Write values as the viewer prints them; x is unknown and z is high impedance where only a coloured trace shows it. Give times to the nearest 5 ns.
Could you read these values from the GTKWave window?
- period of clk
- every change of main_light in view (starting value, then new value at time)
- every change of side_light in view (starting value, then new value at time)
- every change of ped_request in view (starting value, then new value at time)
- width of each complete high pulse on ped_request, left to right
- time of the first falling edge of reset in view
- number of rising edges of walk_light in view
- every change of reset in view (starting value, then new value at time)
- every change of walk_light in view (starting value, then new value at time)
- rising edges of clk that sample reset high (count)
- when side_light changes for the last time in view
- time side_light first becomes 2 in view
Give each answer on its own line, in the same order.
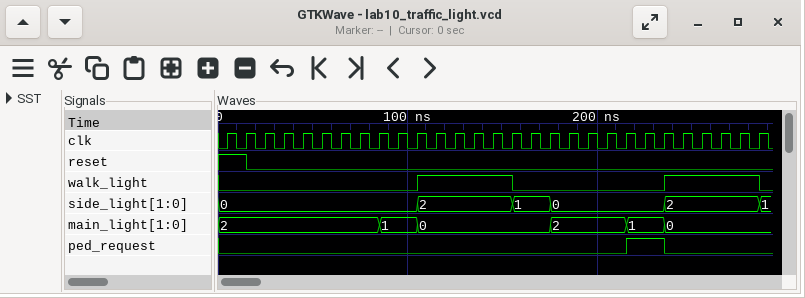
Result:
10 ns
2, 1 at 85 ns, 0 at 105 ns, 2 at 175 ns, 1 at 215 ns, 0 at 235 ns
0, 2 at 105 ns, 1 at 155 ns, 0 at 175 ns, 2 at 235 ns, 1 at 285 ns
0, 1 at 215 ns, 0 at 235 ns
20 ns
15 ns
2
1, 0 at 15 ns
0, 1 at 105 ns, 0 at 155 ns, 1 at 235 ns, 0 at 285 ns
2
285 ns
105 ns
